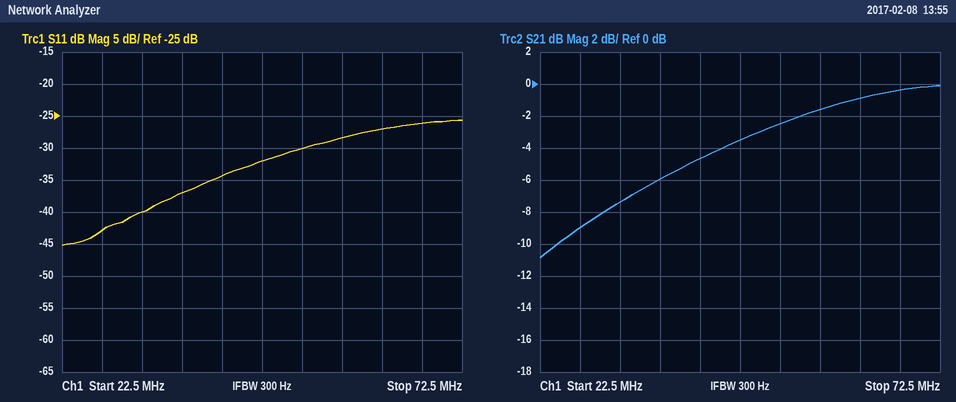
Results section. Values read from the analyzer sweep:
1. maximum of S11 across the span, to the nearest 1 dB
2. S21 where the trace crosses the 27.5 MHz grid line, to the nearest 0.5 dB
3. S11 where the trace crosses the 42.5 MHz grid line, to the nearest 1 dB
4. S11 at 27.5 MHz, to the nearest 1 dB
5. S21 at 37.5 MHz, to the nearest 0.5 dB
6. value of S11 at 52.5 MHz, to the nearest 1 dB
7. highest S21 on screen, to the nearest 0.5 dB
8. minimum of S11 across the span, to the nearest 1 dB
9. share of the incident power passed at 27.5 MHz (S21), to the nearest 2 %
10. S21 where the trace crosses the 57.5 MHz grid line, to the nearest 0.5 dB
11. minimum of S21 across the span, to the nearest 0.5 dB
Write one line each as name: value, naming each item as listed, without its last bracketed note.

maximum of S11 across the span, to the nearest 1 dB: -26 dB
S21 where the trace crosses the 27.5 MHz grid line, to the nearest 0.5 dB: -9.0 dB
S11 where the trace crosses the 42.5 MHz grid line, to the nearest 1 dB: -34 dB
S11 at 27.5 MHz, to the nearest 1 dB: -43 dB
S21 at 37.5 MHz, to the nearest 0.5 dB: -6.0 dB
value of S11 at 52.5 MHz, to the nearest 1 dB: -30 dB
highest S21 on screen, to the nearest 0.5 dB: 0.0 dB
minimum of S11 across the span, to the nearest 1 dB: -45 dB
share of the incident power passed at 27.5 MHz (S21), to the nearest 2 %: 12 %
S21 where the trace crosses the 57.5 MHz grid line, to the nearest 0.5 dB: -1.5 dB
minimum of S21 across the span, to the nearest 0.5 dB: -11.0 dB
